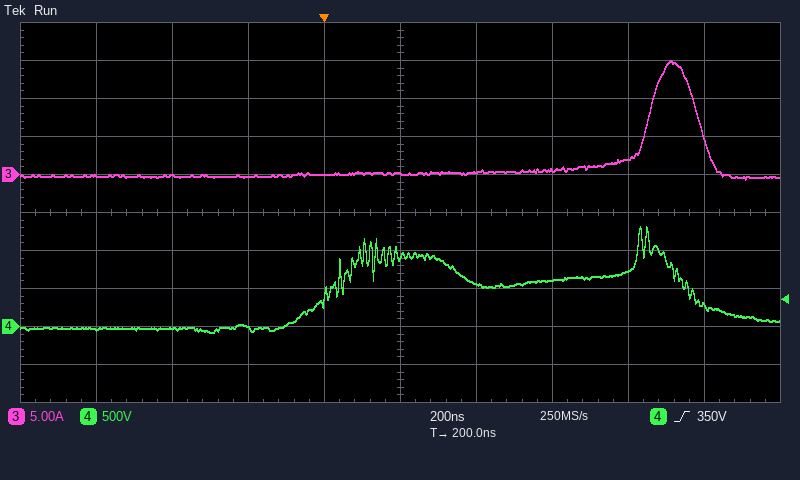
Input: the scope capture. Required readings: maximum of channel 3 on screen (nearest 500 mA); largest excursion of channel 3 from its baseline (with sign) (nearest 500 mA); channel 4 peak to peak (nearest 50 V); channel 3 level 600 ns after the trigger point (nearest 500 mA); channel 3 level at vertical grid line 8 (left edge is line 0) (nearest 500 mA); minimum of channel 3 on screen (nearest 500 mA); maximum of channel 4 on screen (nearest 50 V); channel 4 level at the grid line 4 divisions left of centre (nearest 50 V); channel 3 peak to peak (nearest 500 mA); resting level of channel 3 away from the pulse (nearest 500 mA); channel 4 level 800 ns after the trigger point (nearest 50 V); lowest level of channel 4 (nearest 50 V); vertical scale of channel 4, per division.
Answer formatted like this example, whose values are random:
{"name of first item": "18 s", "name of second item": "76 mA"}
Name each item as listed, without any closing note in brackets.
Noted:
{"maximum of channel 3 on screen": "15.0 A", "largest excursion of channel 3 from its baseline (with sign)": "+15.0 A", "channel 4 peak to peak": "1.40 kV", "channel 3 level 600 ns after the trigger point": "500 mA", "channel 3 level at vertical grid line 8 (left edge is line 0)": "2.0 A", "minimum of channel 3 on screen": "-500 mA", "maximum of channel 4 on screen": "1.30 kV", "channel 4 level at the grid line 4 divisions left of centre": "-50 V", "channel 3 peak to peak": "15.5 A", "resting level of channel 3 away from the pulse": "0.0 A", "channel 4 level 800 ns after the trigger point": "750 V", "lowest level of channel 4": "-100 V", "vertical scale of channel 4, per division": "500 V"}
